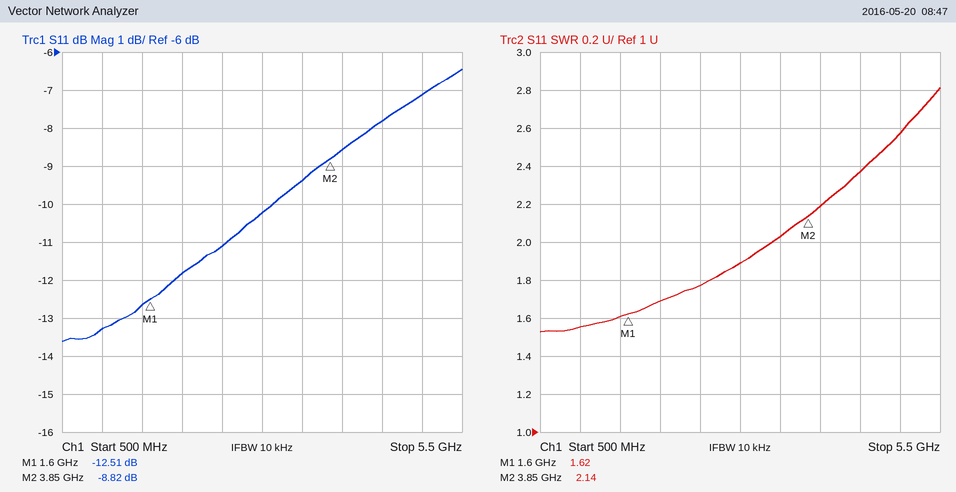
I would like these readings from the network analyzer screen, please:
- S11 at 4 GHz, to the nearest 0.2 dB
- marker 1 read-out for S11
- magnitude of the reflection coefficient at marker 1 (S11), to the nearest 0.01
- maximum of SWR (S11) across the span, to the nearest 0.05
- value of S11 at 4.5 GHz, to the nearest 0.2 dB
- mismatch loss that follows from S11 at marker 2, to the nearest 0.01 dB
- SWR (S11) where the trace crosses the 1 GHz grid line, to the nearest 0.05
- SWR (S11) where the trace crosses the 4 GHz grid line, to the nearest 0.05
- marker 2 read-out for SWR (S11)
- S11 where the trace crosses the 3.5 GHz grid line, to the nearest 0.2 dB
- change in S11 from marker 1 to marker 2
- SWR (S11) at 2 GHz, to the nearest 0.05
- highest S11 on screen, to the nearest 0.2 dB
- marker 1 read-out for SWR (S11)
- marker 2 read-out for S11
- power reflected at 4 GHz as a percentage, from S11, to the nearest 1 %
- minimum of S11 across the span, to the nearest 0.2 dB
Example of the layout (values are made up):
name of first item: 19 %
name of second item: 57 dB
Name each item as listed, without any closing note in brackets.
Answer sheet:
S11 at 4 GHz, to the nearest 0.2 dB: -8.6 dB
marker 1 read-out for S11: -12.51 dB
magnitude of the reflection coefficient at marker 1 (S11), to the nearest 0.01: 0.24
maximum of SWR (S11) across the span, to the nearest 0.05: 2.80
value of S11 at 4.5 GHz, to the nearest 0.2 dB: -7.8 dB
mismatch loss that follows from S11 at marker 2, to the nearest 0.01 dB: 0.61 dB
SWR (S11) where the trace crosses the 1 GHz grid line, to the nearest 0.05: 1.55
SWR (S11) where the trace crosses the 4 GHz grid line, to the nearest 0.05: 2.20
marker 2 read-out for SWR: 2.14
S11 where the trace crosses the 3.5 GHz grid line, to the nearest 0.2 dB: -9.4 dB
change in S11 from marker 1 to marker 2: 3.69 dB
SWR (S11) at 2 GHz, to the nearest 0.05: 1.70
highest S11 on screen, to the nearest 0.2 dB: -6.4 dB
marker 1 read-out for SWR: 1.62
marker 2 read-out for S11: -8.82 dB
power reflected at 4 GHz as a percentage, from S11, to the nearest 1 %: 14 %
minimum of S11 across the span, to the nearest 0.2 dB: -13.6 dB
